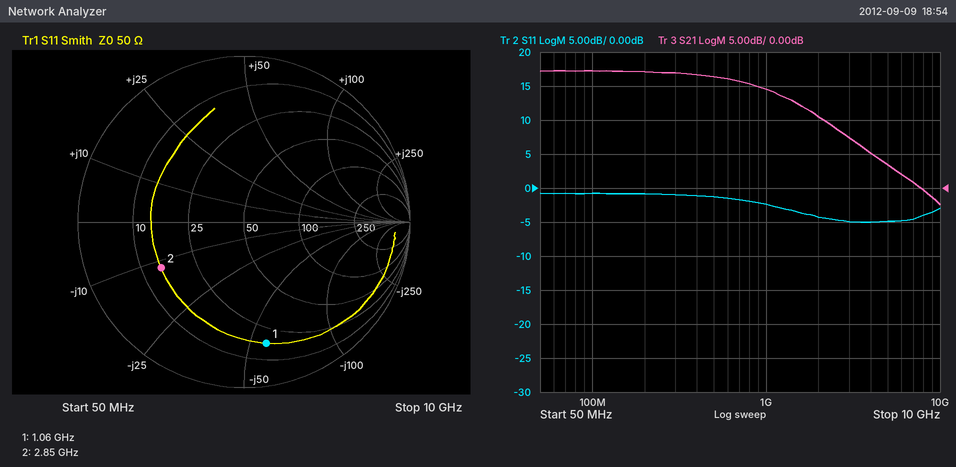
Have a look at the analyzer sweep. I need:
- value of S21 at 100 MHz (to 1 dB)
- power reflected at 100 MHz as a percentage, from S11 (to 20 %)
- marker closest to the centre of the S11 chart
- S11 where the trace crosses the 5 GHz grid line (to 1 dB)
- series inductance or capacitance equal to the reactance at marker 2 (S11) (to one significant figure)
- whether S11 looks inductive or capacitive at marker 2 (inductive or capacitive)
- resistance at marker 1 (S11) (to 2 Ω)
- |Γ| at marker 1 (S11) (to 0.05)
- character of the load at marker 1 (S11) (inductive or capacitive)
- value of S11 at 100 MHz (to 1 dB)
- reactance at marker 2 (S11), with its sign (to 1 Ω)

17 dB
80 %
marker 2
-5 dB
5 pF
capacitive
18 Ω
0.75
capacitive
-1 dB
-12 Ω
